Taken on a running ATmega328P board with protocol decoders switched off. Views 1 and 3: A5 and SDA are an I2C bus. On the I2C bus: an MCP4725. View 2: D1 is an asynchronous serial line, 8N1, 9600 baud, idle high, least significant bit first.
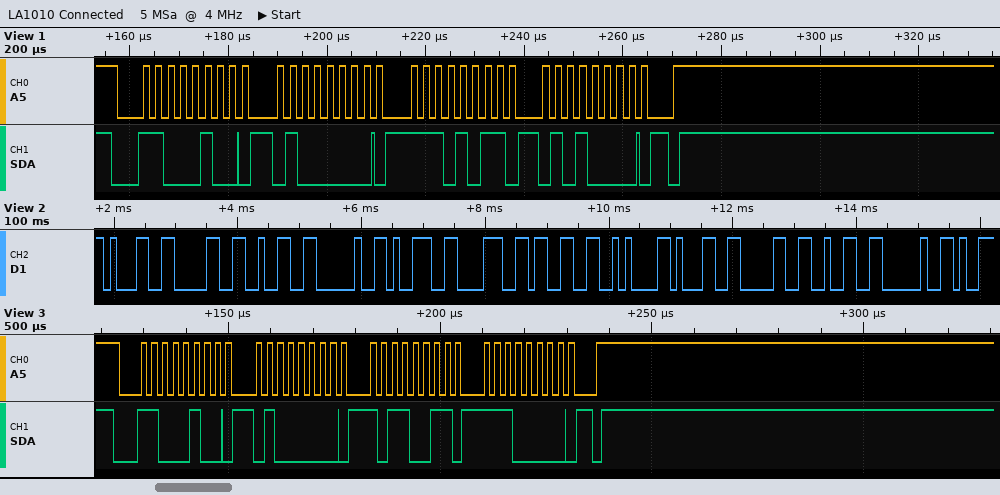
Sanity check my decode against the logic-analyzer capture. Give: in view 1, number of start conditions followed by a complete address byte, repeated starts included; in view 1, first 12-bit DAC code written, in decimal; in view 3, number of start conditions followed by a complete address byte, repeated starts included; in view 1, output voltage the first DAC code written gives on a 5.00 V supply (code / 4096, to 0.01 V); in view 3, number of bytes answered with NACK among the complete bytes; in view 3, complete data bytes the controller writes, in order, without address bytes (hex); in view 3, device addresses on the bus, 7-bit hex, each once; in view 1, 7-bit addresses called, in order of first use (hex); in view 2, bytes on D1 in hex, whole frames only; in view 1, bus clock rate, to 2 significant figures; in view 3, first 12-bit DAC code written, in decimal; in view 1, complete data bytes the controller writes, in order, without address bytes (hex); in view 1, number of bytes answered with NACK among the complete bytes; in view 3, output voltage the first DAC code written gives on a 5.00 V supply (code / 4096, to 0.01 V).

1
3765
1
4.60 V
0
40 B3 E0
0x62
0x62
31 30 32 20 39 38 33 0A 31 30 32 20
400 kHz
2878
40 EB 50
0
3.51 V
